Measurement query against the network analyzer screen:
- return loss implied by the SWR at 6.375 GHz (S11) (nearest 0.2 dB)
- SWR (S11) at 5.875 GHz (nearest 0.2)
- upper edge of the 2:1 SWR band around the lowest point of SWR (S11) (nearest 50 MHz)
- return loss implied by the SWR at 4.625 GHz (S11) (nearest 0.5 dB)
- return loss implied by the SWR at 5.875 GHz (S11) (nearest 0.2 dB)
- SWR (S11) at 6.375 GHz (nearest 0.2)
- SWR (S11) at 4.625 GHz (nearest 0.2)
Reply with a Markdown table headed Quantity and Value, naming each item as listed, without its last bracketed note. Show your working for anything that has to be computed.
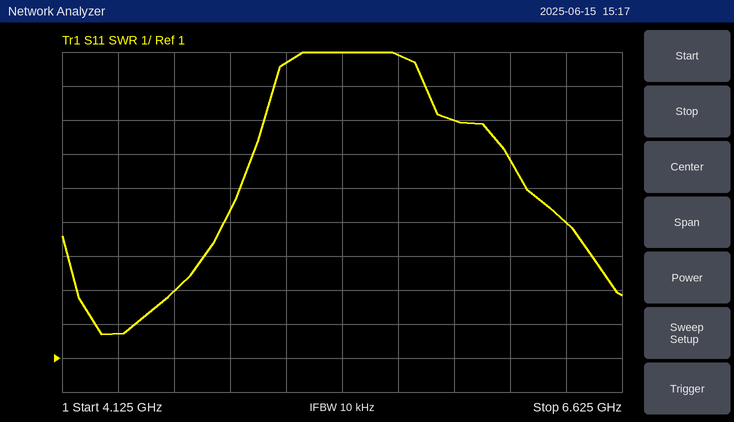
| Quantity | Value |
|---|---|
| return loss implied by the SWR at 6.375 GHz (S11) | −20 log10((5 − 1)/(5 + 1)) ≈ 3.52 dB, so 3.6 dB to the nearest 0.2 dB |
| SWR (S11) at 5.875 GHz | 8.0 |
| upper edge of the 2:1 SWR band around the lowest point of SWR (S11) | 4.45 GHz |
| return loss implied by the SWR at 4.625 GHz (S11) | −20 log10((3 − 1)/(3 + 1)) ≈ 6.0 dB |
| return loss implied by the SWR at 5.875 GHz (S11) | −20 log10((8 − 1)/(8 + 1)) ≈ 2.2 dB |
| SWR (S11) at 6.375 GHz | 5.0 |
| SWR (S11) at 4.625 GHz | 3.0 |
